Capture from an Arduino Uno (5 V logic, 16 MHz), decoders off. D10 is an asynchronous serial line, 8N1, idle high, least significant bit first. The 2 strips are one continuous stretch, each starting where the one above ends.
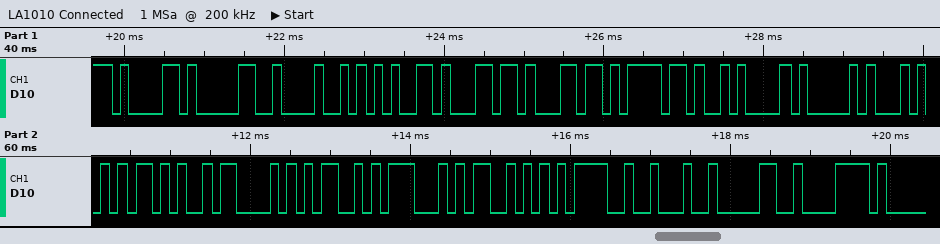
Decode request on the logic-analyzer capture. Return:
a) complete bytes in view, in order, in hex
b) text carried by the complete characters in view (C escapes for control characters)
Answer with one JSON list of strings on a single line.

["0x61 0x30 0x48 0x65 0x6C 0x6C 0x6F 0x0A 0x41 0x54 0x2B 0x43 0x4D 0x47 0x53 0x3D 0x22 0x30 0x78", "\"a0Hello\\nAT+CMGS=\\\"0x\""]
